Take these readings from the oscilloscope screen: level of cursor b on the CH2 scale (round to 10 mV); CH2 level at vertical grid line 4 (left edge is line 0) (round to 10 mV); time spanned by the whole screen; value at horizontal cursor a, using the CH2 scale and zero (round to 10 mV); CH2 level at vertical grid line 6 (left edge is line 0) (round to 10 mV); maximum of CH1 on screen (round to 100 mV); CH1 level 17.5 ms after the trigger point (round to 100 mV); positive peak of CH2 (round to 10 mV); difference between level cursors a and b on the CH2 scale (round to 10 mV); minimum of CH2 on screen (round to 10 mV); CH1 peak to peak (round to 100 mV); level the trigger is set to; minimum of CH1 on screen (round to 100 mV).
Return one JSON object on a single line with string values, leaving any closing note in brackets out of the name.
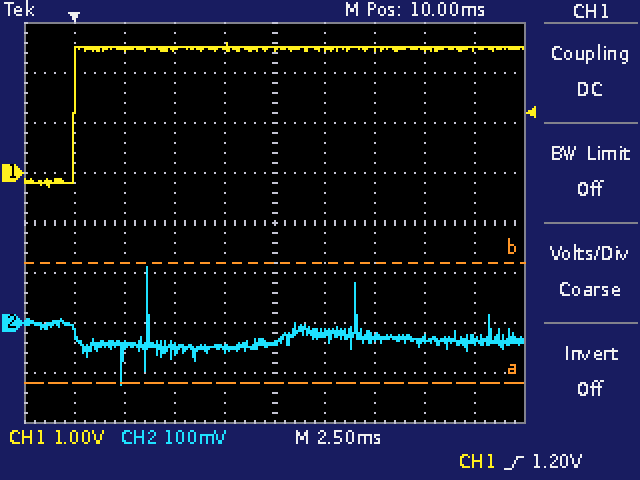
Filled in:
{"level of cursor b on the CH2 scale": "120 mV", "CH2 level at vertical grid line 4 (left edge is line 0)": "-50 mV", "time spanned by the whole screen": "25 ms", "value at horizontal cursor a, using the CH2 scale and zero": "-120 mV", "CH2 level at vertical grid line 6 (left edge is line 0)": "-20 mV", "maximum of CH1 on screen": "2.6 V", "CH1 level 17.5 ms after the trigger point": "2.5 V", "positive peak of CH2": "110 mV", "difference between level cursors a and b on the CH2 scale": "240 mV", "minimum of CH2 on screen": "-120 mV", "CH1 peak to peak": "2.9 V", "level the trigger is set to": "1.20 V", "minimum of CH1 on screen": "-300 mV"}
